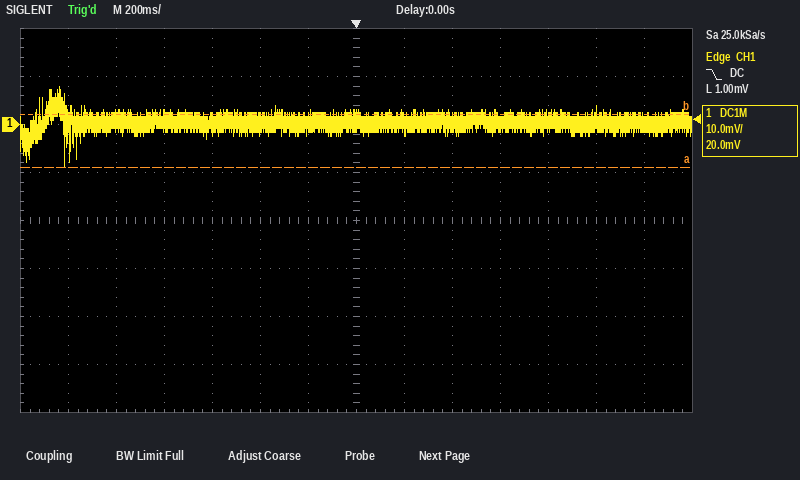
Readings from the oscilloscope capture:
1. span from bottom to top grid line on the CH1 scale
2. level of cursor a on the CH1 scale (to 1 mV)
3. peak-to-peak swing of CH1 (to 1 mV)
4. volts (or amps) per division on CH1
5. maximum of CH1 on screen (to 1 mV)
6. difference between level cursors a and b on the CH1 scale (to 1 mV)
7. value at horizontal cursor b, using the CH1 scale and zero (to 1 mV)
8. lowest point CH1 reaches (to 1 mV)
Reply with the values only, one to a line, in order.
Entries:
80 mV
-9 mV
17 mV
10 mV
8 mV
11 mV
2 mV
-9 mV
